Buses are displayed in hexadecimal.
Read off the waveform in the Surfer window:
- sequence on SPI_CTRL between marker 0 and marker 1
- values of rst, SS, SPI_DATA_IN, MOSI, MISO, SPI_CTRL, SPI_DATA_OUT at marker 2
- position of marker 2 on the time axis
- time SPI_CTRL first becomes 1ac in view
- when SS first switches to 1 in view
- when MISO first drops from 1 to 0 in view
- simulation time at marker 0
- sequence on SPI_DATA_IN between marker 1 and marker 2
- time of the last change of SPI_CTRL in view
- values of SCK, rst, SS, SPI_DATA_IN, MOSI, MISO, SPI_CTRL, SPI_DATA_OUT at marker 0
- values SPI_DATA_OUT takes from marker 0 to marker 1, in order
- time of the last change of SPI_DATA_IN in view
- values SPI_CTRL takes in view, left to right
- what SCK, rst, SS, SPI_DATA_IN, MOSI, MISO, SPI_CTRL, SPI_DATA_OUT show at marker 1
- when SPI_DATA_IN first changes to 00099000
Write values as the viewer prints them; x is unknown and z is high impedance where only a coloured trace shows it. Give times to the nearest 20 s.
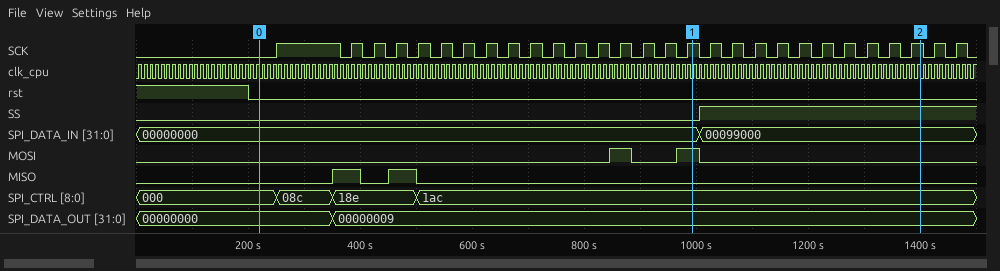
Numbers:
000, 08c, 18e, 1ac
rst=0, SS=1, SPI_DATA_IN=00099000, MOSI=0, MISO=0, SPI_CTRL=1ac, SPI_DATA_OUT=00000009
1400 s
500 s
1000 s
400 s
220 s
00000000, 00099000
500 s
SCK=0, rst=0, SS=0, SPI_DATA_IN=00000000, MOSI=0, MISO=0, SPI_CTRL=000, SPI_DATA_OUT=00000000
00000000, 00000009
1000 s
000, 08c, 18e, 1ac
SCK=1, rst=0, SS=0, SPI_DATA_IN=00000000, MOSI=1, MISO=0, SPI_CTRL=1ac, SPI_DATA_OUT=00000009
1000 s
